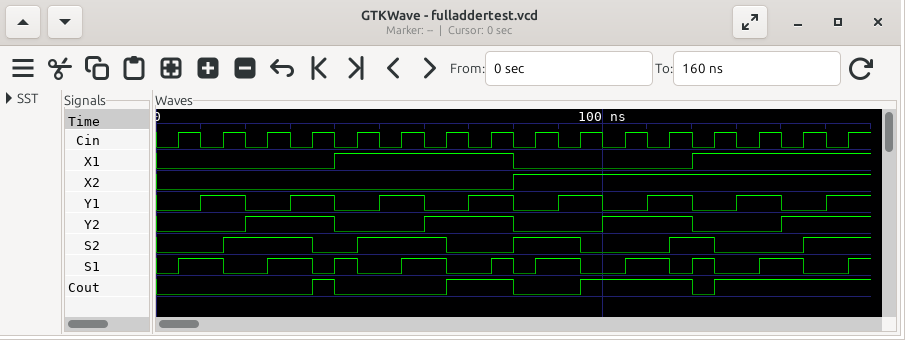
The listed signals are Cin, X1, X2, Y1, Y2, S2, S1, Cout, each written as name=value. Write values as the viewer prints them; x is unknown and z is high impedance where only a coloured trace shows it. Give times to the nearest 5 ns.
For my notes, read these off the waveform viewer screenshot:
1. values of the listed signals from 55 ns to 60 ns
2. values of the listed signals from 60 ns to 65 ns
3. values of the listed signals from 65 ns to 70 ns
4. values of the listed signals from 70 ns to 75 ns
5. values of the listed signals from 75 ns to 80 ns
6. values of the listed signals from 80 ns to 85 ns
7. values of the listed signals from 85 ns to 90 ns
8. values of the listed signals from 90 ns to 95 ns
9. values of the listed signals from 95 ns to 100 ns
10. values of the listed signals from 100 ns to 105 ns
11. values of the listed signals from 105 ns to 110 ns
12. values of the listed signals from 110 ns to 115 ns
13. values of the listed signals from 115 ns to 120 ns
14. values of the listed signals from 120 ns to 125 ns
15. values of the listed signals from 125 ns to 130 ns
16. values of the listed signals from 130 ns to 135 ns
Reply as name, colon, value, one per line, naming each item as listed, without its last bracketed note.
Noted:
values of the listed signals from 55 ns to 60 ns: Cin=1, X1=1, X2=0, Y1=1, Y2=0, S2=1, S1=1, Cout=0
values of the listed signals from 60 ns to 65 ns: Cin=0, X1=1, X2=0, Y1=0, Y2=1, S2=1, S1=1, Cout=0
values of the listed signals from 65 ns to 70 ns: Cin=1, X1=1, X2=0, Y1=0, Y2=1, S2=0, S1=0, Cout=1
values of the listed signals from 70 ns to 75 ns: Cin=0, X1=1, X2=0, Y1=1, Y2=1, S2=0, S1=0, Cout=1
values of the listed signals from 75 ns to 80 ns: Cin=1, X1=1, X2=0, Y1=1, Y2=1, S2=0, S1=1, Cout=1
values of the listed signals from 80 ns to 85 ns: Cin=0, X1=0, X2=1, Y1=0, Y2=0, S2=1, S1=0, Cout=0
values of the listed signals from 85 ns to 90 ns: Cin=1, X1=0, X2=1, Y1=0, Y2=0, S2=1, S1=1, Cout=0
values of the listed signals from 90 ns to 95 ns: Cin=0, X1=0, X2=1, Y1=1, Y2=0, S2=1, S1=1, Cout=0
values of the listed signals from 95 ns to 100 ns: Cin=1, X1=0, X2=1, Y1=1, Y2=0, S2=0, S1=0, Cout=1
values of the listed signals from 100 ns to 105 ns: Cin=0, X1=0, X2=1, Y1=0, Y2=1, S2=0, S1=0, Cout=1
values of the listed signals from 105 ns to 110 ns: Cin=1, X1=0, X2=1, Y1=0, Y2=1, S2=0, S1=1, Cout=1
values of the listed signals from 110 ns to 115 ns: Cin=0, X1=0, X2=1, Y1=1, Y2=1, S2=0, S1=1, Cout=1
values of the listed signals from 115 ns to 120 ns: Cin=1, X1=0, X2=1, Y1=1, Y2=1, S2=1, S1=0, Cout=1
values of the listed signals from 120 ns to 125 ns: Cin=0, X1=1, X2=1, Y1=0, Y2=0, S2=1, S1=1, Cout=0
values of the listed signals from 125 ns to 130 ns: Cin=1, X1=1, X2=1, Y1=0, Y2=0, S2=0, S1=0, Cout=1
values of the listed signals from 130 ns to 135 ns: Cin=0, X1=1, X2=1, Y1=1, Y2=0, S2=0, S1=0, Cout=1
